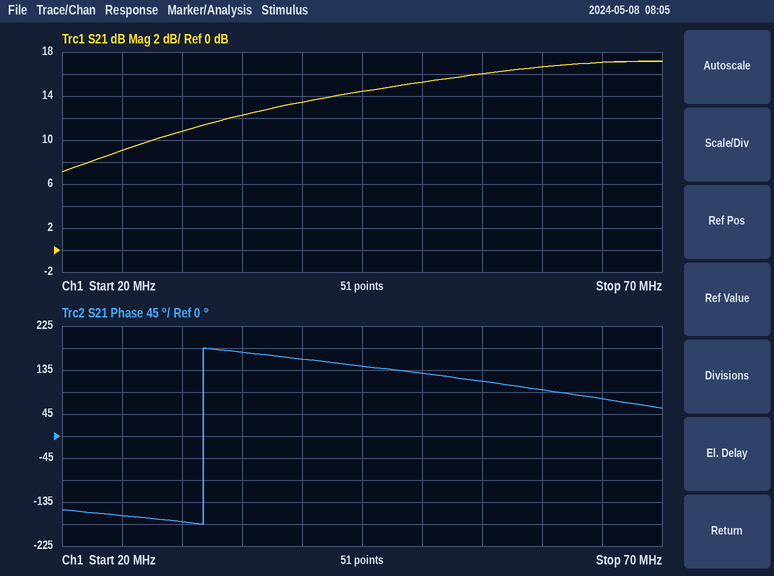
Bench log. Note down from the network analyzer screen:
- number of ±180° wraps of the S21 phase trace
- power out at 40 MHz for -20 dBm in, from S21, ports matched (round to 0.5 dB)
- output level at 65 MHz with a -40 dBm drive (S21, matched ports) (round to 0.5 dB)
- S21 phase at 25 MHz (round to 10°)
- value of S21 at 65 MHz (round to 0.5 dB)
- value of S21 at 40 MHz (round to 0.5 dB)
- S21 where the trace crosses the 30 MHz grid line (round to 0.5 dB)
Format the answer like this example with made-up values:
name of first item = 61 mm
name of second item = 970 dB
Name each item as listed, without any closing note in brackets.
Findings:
number of ±180° wraps of the S21 phase trace = 1
power out at 40 MHz for -20 dBm in, from S21, ports matched = -6.5 dBm
output level at 65 MHz with a -40 dBm drive (S21, matched ports) = -23.0 dBm
S21 phase at 25 MHz = -160°
value of S21 at 65 MHz = 17.0 dB
value of S21 at 40 MHz = 13.5 dB
S21 where the trace crosses the 30 MHz grid line = 11.0 dB
